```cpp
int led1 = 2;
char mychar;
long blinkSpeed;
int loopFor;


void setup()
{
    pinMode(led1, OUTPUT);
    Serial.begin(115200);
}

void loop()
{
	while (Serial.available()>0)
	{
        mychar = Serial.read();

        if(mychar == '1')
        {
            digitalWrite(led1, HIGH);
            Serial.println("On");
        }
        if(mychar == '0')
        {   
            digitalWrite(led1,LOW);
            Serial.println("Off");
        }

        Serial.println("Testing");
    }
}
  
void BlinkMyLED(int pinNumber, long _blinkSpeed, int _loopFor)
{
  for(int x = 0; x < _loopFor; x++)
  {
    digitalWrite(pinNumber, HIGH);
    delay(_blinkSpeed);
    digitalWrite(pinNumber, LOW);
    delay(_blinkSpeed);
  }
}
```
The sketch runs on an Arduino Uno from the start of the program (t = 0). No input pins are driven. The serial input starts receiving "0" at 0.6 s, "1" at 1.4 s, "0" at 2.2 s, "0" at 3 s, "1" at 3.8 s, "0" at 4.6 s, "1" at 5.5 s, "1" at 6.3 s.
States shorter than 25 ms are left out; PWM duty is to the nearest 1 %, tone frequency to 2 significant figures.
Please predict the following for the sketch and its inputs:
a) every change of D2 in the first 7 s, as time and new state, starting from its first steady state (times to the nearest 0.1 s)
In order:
0 s low; 1.4 s high; 2.2 s low; 3.8 s high; 4.6 s low; 5.5 s high
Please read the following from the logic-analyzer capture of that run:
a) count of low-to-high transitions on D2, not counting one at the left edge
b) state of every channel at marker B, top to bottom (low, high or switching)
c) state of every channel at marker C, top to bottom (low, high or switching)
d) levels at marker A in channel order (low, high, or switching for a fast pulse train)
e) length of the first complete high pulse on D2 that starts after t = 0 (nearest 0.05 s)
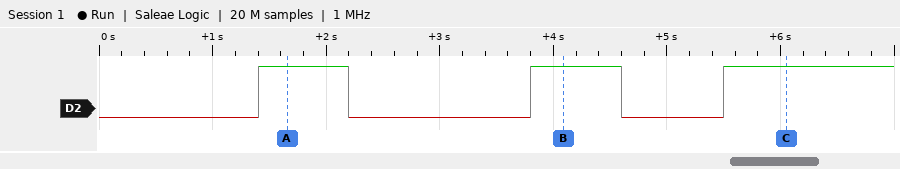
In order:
3
D2 high
D2 high
D2 high
0.80 s
